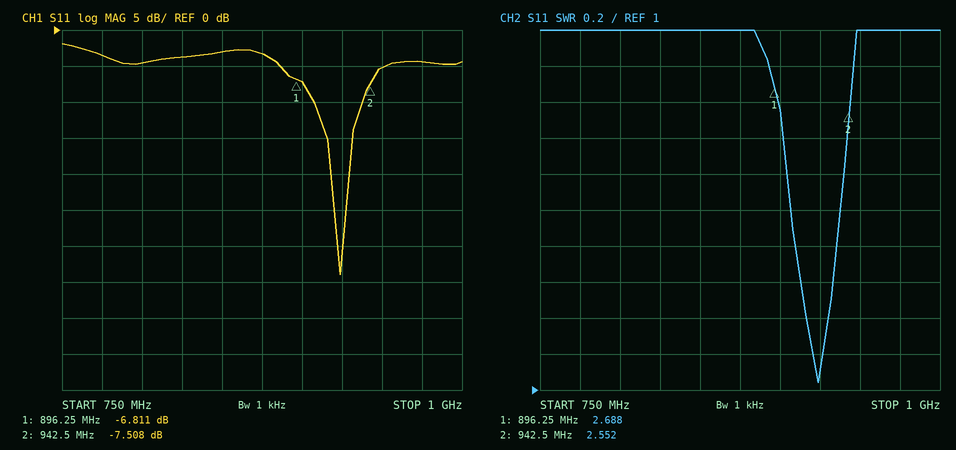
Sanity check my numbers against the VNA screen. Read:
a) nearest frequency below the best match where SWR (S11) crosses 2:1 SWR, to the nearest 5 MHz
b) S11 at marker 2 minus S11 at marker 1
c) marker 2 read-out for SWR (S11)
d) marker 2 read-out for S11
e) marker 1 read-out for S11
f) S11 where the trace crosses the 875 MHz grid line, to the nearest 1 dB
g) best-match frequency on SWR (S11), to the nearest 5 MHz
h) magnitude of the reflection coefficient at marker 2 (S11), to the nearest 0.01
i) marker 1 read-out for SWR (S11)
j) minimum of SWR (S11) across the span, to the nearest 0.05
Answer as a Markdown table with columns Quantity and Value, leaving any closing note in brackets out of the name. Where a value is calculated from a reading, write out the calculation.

| Quantity | Value |
|---|---|
| nearest frequency below the best match where SWR (S11) crosses 2:1 SWR, to the nearest 5 MHz | 905 MHz |
| S11 at marker 2 minus S11 at marker 1 | -7.508 − (-6.811) = -0.697 dB |
| marker 2 read-out for SWR | 2.552 |
| marker 2 read-out for S11 | -7.508 dB |
| marker 1 read-out for S11 | -6.811 dB |
| S11 where the trace crosses the 875 MHz grid line, to the nearest 1 dB | -3 dB |
| best-match frequency on SWR (S11), to the nearest 5 MHz | 925 MHz |
| magnitude of the reflection coefficient at marker 2 (S11), to the nearest 0.01 | 10^(-7.508/20) ≈ 0.42 |
| marker 1 read-out for SWR | 2.688 |
| minimum of SWR (S11) across the span, to the nearest 0.05 | 1.05 |
